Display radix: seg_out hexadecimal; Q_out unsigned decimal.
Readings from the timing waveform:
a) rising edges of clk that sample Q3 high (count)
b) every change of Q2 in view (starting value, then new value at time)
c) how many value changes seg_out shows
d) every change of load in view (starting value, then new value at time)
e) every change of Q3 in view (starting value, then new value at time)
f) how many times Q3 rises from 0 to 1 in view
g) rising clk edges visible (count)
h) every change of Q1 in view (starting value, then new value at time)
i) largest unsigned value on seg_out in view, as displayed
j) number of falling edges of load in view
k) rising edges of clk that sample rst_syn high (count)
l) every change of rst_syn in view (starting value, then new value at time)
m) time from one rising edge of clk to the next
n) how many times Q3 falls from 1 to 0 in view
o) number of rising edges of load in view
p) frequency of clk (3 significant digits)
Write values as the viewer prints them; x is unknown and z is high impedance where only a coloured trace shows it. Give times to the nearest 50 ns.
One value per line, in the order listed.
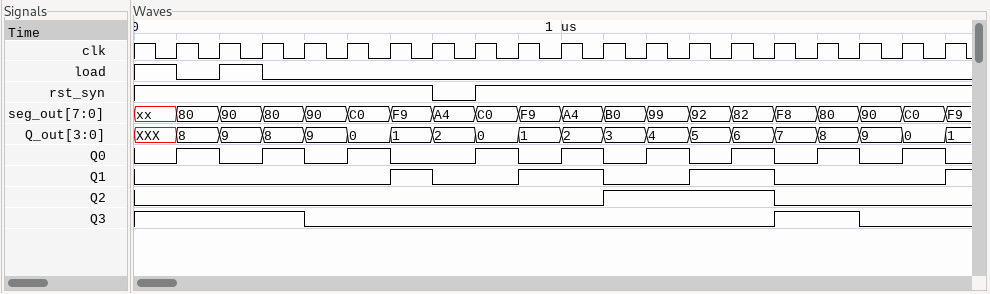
6
0, 1 at 1100 ns, 0 at 1500 ns
19
1, 0 at 100 ns, 1 at 200 ns, 0 at 300 ns
1, 0 at 400 ns, 1 at 1500 ns, 0 at 1700 ns
1
19
0, 1 at 600 ns, 0 at 700 ns, 1 at 900 ns, 0 at 1100 ns, 1 at 1300 ns, 0 at 1500 ns, 1 at 1900 ns
F9
2
18
1, 0 at 700 ns, 1 at 800 ns
100 ns
2
1
10.0 MHz
